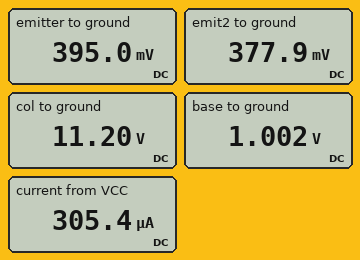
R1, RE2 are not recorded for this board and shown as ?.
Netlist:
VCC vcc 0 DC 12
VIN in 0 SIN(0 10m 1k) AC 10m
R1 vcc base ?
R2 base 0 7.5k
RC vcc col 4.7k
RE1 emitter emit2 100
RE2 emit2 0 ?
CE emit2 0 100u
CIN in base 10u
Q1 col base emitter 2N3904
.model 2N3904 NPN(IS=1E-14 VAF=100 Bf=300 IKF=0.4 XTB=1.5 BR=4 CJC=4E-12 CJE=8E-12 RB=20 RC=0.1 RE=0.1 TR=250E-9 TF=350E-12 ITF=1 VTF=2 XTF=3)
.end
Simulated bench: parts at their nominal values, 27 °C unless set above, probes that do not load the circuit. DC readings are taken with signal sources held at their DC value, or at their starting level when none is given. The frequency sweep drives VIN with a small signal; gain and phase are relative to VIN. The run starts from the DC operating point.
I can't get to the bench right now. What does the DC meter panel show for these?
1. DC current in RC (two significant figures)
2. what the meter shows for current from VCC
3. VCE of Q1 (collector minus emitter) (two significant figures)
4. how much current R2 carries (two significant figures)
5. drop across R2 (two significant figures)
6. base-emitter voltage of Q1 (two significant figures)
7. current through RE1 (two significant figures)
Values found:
170 µA
305.4 µA
11 V
130 µA
1.0 V
610 mV
170 µA
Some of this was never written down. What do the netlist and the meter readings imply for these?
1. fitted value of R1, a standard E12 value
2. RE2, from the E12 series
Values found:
82 kΩ
2.2 kΩ
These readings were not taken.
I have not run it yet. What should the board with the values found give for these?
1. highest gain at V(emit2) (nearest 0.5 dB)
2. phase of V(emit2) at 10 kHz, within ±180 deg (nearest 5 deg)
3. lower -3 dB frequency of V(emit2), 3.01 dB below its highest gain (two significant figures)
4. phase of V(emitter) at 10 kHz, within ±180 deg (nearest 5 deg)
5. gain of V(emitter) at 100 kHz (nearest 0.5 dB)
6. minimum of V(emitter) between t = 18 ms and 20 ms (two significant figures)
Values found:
-3.5 dB
-90 deg
1.5 Hz
0 deg
-8.0 dB
390 mV
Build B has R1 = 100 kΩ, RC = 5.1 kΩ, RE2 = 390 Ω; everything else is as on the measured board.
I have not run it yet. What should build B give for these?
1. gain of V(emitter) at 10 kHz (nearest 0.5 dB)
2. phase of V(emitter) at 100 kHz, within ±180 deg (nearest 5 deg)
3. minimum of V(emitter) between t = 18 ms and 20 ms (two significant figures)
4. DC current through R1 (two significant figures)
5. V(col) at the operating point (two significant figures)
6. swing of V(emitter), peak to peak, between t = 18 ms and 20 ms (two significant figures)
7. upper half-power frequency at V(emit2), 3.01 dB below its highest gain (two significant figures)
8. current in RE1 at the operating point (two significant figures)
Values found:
-4.5 dB
0 deg
190 mV
110 µA
9.9 V
12 mV
18 Hz
410 µA
